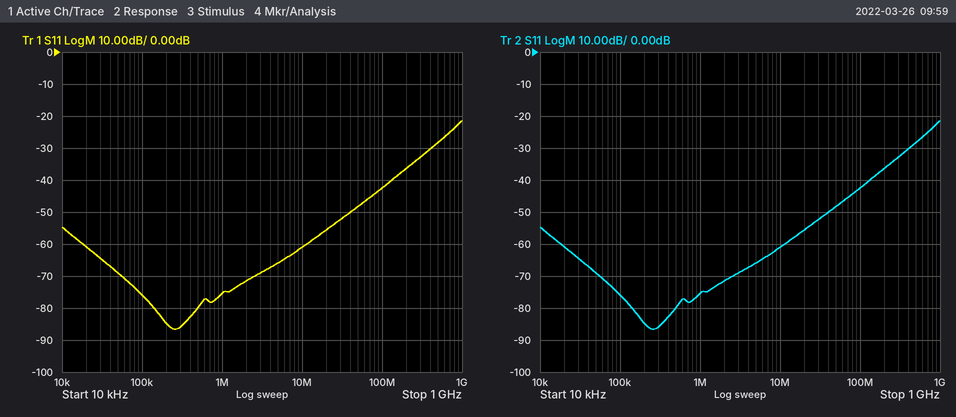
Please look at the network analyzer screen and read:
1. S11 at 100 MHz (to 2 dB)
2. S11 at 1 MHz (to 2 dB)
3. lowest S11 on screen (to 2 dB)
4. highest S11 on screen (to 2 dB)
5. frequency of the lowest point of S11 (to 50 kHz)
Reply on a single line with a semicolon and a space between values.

-42 dB; -76 dB; -86 dB; -22 dB; 250 kHz
